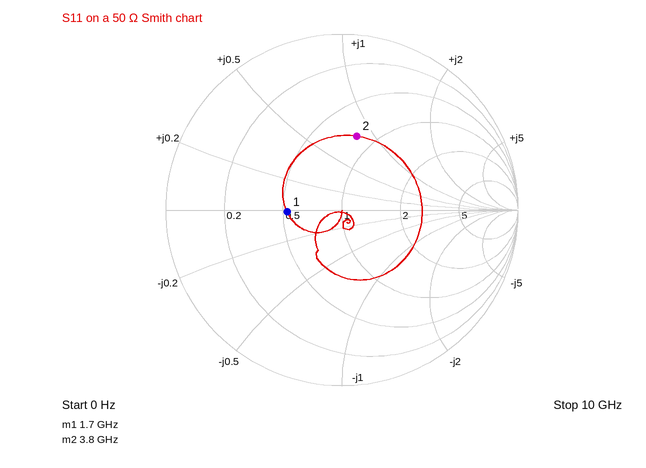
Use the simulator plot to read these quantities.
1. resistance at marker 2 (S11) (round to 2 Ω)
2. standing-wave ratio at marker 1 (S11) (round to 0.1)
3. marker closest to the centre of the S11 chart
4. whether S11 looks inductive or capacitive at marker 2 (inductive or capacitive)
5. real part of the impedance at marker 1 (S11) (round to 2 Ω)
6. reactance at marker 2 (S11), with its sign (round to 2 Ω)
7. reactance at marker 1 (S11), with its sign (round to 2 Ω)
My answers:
40 Ω
1.9
marker 1
inductive
26 Ω
+42 Ω
0 Ω
